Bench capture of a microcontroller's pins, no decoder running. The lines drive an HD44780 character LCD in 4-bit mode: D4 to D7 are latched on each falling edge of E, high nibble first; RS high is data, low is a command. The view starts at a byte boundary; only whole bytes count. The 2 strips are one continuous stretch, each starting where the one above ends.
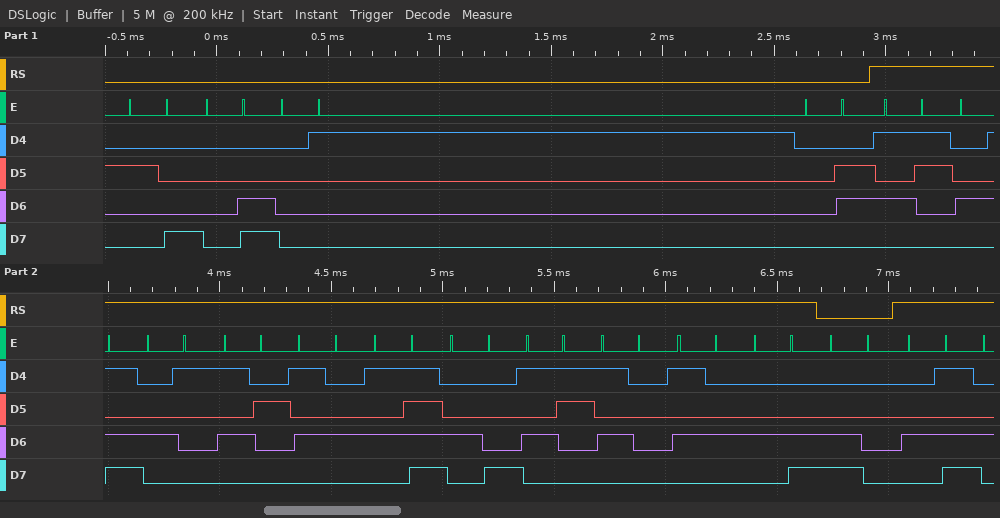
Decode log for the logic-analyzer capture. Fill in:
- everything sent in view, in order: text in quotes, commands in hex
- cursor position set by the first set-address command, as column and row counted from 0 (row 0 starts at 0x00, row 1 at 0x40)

0x28 0x0C 0x01 0x06 "SMART_HSPTL" 0xC0 "M"
column 0, row 1
